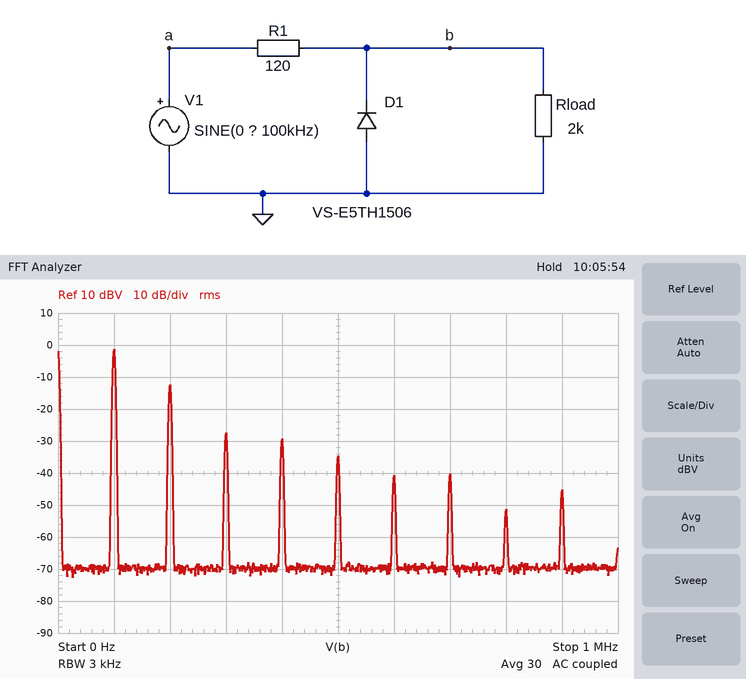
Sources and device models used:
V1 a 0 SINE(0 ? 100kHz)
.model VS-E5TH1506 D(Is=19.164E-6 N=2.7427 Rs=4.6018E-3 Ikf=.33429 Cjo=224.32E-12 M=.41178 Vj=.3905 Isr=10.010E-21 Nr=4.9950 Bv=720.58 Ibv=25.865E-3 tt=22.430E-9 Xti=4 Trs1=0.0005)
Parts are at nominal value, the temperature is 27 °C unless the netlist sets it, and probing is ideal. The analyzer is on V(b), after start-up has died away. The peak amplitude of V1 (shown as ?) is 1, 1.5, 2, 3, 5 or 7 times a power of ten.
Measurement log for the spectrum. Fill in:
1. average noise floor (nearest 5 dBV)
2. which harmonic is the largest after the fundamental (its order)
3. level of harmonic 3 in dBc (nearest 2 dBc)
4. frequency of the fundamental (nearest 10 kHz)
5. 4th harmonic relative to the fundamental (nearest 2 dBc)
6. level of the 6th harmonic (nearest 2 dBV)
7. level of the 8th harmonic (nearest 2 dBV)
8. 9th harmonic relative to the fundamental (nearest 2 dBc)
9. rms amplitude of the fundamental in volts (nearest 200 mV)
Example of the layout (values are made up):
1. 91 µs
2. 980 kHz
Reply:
1. -70 dBV
2. 2
3. -26 dBc
4. 100 kHz
5. -28 dBc
6. -40 dBV
7. -52 dBV
8. -44 dBc
9. 800 mV
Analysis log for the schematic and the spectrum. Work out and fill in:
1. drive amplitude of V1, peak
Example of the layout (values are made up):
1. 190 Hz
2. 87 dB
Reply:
1. 2 V
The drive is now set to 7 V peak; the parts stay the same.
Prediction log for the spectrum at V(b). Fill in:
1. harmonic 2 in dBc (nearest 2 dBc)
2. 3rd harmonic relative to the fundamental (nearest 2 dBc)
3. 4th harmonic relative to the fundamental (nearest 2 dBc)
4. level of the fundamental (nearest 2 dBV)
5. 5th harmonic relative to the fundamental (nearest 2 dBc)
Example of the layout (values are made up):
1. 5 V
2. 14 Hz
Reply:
1. -8 dBc
2. -32 dBc
3. -24 dBc
4. 8 dBV
5. -38 dBc
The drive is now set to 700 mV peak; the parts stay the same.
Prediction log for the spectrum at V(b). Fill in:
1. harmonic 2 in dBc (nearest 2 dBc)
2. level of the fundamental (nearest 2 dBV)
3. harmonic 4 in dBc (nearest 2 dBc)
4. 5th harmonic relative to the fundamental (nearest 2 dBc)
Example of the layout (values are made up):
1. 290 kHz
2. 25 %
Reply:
1. -16 dBc
2. -8 dBV
3. -52 dBc
4. -40 dBc
